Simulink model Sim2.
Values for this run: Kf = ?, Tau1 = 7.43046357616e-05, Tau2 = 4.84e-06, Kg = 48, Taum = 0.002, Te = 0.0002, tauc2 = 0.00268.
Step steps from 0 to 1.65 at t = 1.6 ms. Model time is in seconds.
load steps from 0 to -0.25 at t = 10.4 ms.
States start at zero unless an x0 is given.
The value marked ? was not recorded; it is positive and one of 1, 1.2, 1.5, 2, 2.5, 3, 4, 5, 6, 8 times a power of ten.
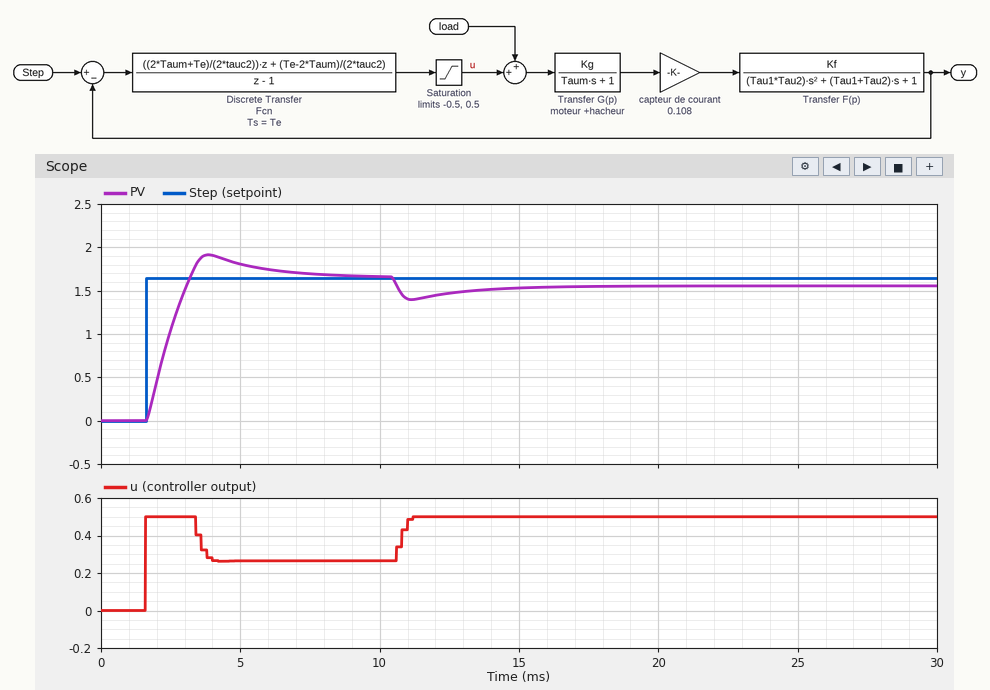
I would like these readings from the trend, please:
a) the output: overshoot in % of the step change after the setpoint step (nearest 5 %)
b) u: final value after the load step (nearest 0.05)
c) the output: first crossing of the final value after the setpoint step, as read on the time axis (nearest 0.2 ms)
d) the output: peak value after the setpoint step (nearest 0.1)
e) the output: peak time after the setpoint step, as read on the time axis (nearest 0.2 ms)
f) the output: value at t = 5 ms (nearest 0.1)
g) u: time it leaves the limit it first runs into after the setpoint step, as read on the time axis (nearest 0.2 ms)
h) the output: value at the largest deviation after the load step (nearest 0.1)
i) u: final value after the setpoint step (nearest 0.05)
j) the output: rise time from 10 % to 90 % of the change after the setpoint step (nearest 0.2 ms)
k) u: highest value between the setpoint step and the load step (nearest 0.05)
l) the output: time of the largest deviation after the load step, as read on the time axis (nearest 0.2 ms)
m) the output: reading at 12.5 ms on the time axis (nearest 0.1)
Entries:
15 %
0.50
3.2 ms
1.9
3.8 ms
1.8
3.4 ms
1.4
0.25
1.2 ms
0.50
11.2 ms
1.5
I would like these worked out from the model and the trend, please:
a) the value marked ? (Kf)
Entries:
1.2
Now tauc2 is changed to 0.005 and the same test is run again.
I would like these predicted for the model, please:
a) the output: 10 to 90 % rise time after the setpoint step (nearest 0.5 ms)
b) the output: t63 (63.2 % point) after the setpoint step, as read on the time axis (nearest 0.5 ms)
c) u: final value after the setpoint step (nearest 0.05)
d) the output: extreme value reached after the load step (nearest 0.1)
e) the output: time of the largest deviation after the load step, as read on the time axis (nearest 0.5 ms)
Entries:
1.5 ms
2.5 ms
0.25
1.3
11.5 ms
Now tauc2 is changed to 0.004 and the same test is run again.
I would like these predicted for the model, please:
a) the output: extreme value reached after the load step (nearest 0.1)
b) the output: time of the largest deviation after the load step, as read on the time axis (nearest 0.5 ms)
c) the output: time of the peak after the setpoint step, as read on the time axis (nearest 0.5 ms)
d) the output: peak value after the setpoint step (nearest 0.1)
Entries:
1.3
11.5 ms
4.0 ms
1.8
